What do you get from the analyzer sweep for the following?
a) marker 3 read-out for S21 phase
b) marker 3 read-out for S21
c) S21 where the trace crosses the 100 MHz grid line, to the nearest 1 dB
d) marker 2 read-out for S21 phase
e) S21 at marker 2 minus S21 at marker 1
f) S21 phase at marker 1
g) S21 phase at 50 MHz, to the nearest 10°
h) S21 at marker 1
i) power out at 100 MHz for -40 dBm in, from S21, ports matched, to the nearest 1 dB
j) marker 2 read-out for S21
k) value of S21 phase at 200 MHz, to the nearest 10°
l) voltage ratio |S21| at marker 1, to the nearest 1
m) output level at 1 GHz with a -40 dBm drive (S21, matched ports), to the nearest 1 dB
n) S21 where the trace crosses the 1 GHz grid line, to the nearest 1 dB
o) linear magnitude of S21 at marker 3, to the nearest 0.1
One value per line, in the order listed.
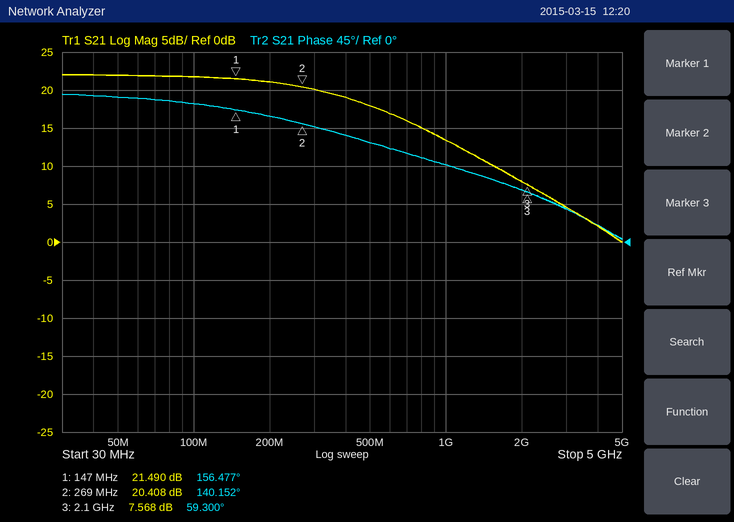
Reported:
59.300°
7.568 dB
22 dB
140.152°
-1.082 dB
156.477°
170°
21.490 dB
-18 dBm
20.408 dB
150°
12
-27 dBm
13 dB
2.4
